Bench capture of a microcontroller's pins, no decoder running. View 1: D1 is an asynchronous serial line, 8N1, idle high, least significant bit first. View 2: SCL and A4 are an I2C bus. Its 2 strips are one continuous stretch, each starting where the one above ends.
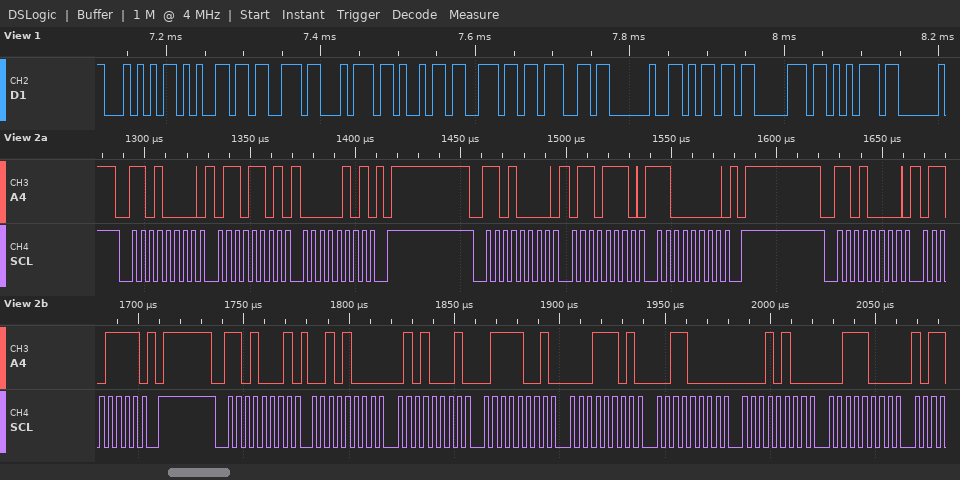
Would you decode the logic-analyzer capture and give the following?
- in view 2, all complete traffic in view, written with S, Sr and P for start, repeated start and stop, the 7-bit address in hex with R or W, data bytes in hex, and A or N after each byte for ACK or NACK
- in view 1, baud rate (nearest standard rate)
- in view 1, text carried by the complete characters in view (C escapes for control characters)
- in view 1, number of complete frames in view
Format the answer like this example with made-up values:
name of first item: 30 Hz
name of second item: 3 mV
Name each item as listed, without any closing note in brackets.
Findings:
in view 2, all complete traffic in view, written with S, Sr and P for start, repeated start and stop, the 7-bit address in hex with R or W, data bytes in hex, and A or N after each byte for ACK or NACK: S 68W A 6D A 05 A P S 68W A 6E A C0 A P S 68W A 6F A P S 68R A 28 A 51 A 79 A 1D A 30 A 14 A 38 A
in view 1, baud rate: 115200 baud
in view 1, text carried by the complete characters in view: "Testing mpu"
in view 1, number of complete frames in view: 11
